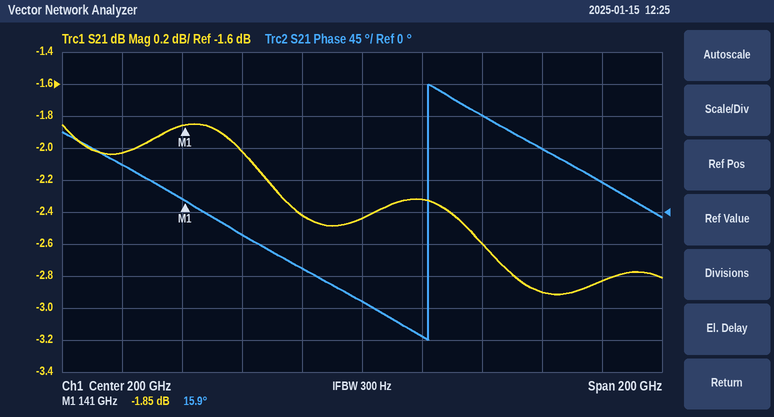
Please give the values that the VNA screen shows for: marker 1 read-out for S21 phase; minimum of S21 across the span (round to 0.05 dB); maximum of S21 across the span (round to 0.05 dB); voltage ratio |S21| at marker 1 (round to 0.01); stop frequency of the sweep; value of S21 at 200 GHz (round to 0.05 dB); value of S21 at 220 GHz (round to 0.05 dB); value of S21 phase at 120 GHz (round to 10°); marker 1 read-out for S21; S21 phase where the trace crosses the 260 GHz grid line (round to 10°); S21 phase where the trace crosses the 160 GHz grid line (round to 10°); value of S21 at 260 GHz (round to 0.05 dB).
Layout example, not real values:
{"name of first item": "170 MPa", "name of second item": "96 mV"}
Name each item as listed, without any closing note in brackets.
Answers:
{"marker 1 read-out for S21 phase": "15.9°", "minimum of S21 across the span": "-2.90 dB", "maximum of S21 across the span": "-1.85 dB", "voltage ratio |S21| at marker 1": "0.81", "stop frequency of the sweep": "300 GHz", "value of S21 at 200 GHz": "-2.45 dB", "value of S21 at 220 GHz": "-2.30 dB", "value of S21 phase at 120 GHz": "70°", "marker 1 read-out for S21": "-1.85 dB", "S21 phase where the trace crosses the 260 GHz grid line": "90°", "S21 phase where the trace crosses the 160 GHz grid line": "-30°", "value of S21 at 260 GHz": "-2.90 dB"}
